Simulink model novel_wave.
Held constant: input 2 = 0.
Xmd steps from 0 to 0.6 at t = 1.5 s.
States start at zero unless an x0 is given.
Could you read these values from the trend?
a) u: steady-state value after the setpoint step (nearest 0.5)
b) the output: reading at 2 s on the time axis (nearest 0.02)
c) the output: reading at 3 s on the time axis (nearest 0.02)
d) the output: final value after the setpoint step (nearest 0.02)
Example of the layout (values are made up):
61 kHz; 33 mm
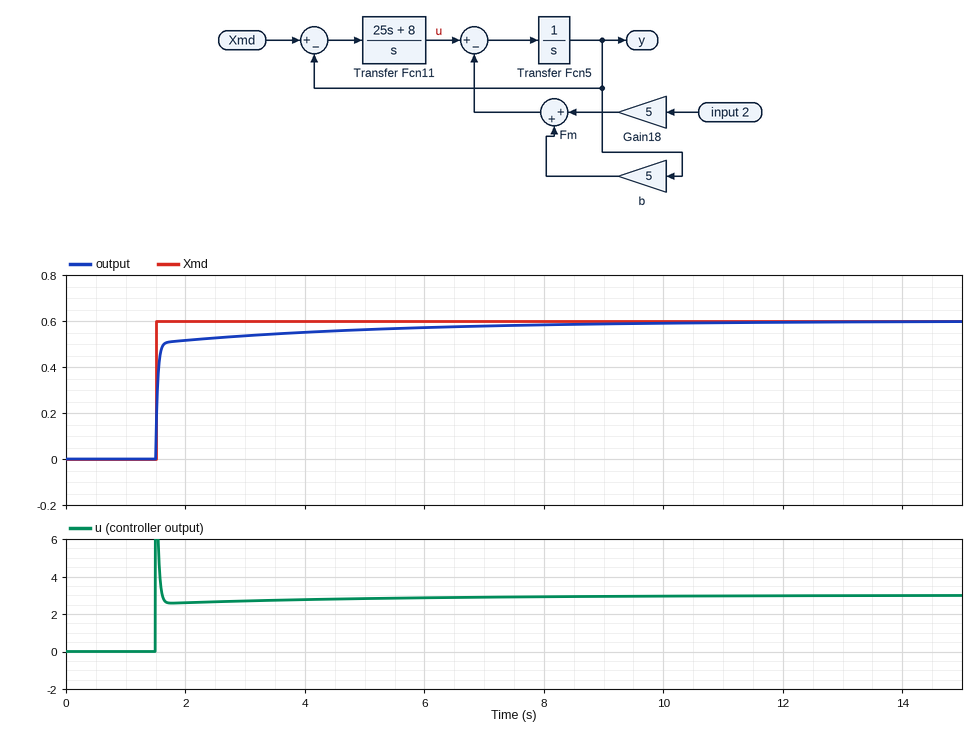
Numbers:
3.0; 0.52; 0.54; 0.60
